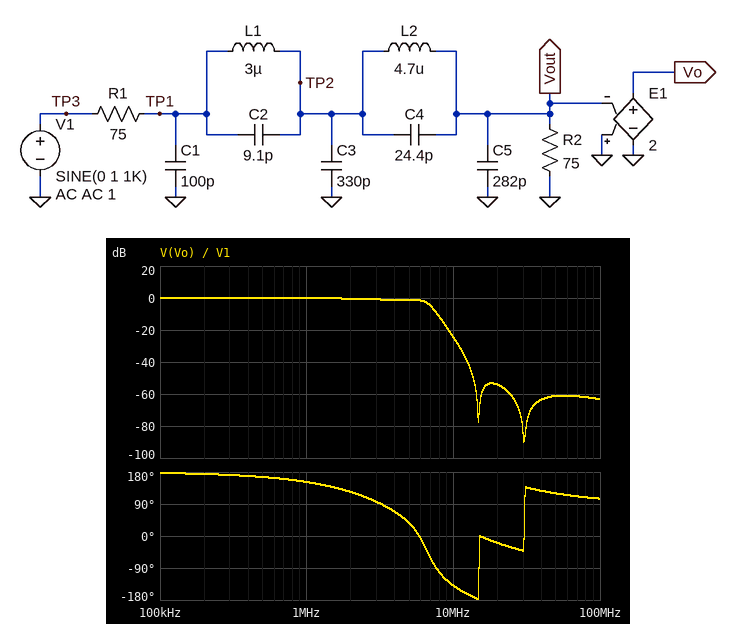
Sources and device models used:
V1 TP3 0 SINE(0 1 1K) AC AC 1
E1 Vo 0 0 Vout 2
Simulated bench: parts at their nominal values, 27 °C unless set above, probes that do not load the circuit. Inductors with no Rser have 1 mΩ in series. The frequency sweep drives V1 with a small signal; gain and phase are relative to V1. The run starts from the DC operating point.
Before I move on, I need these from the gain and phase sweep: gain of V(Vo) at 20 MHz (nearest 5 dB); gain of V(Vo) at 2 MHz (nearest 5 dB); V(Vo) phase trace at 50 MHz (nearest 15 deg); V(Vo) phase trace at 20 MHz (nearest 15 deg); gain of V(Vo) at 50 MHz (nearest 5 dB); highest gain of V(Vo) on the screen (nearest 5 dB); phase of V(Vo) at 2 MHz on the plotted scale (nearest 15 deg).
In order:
-55 dB
0 dB
120 deg
-15 deg
-60 dB
0 dB
120 deg
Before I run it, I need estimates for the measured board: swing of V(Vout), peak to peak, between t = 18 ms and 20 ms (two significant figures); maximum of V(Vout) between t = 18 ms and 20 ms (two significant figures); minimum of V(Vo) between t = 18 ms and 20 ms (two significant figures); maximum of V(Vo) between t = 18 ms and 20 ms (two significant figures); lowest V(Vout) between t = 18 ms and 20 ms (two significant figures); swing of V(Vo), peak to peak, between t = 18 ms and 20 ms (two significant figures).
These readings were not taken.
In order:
1.0 V
500 mV
-1.0 V
1.0 V
-500 mV
2.0 V
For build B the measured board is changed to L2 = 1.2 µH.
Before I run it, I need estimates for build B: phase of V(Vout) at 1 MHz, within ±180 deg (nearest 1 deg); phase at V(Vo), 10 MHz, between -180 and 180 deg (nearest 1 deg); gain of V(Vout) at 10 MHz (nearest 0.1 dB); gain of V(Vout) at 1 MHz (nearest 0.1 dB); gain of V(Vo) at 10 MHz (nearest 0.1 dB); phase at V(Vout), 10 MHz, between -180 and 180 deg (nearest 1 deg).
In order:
-20 deg
-32 deg
-8.7 dB
-6.0 dB
-2.7 dB
148 deg
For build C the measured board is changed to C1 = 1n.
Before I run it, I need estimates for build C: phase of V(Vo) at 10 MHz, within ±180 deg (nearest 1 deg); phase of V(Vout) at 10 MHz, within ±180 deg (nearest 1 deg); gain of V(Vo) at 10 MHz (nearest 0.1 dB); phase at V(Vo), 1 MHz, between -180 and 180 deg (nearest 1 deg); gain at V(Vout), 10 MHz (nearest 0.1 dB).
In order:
144 deg
-36 deg
-37.2 dB
139 deg
-43.2 dB
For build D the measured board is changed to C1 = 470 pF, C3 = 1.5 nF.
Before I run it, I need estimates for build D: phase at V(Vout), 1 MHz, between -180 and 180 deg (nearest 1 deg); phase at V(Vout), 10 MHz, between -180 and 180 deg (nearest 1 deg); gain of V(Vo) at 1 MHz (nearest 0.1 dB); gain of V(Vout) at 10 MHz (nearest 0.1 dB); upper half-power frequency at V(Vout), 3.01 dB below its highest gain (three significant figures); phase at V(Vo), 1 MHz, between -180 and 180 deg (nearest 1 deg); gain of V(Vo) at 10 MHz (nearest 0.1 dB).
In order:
-49 deg
-21 deg
-0.2 dB
-52.7 dB
3.60 MHz
131 deg
-46.7 dB
